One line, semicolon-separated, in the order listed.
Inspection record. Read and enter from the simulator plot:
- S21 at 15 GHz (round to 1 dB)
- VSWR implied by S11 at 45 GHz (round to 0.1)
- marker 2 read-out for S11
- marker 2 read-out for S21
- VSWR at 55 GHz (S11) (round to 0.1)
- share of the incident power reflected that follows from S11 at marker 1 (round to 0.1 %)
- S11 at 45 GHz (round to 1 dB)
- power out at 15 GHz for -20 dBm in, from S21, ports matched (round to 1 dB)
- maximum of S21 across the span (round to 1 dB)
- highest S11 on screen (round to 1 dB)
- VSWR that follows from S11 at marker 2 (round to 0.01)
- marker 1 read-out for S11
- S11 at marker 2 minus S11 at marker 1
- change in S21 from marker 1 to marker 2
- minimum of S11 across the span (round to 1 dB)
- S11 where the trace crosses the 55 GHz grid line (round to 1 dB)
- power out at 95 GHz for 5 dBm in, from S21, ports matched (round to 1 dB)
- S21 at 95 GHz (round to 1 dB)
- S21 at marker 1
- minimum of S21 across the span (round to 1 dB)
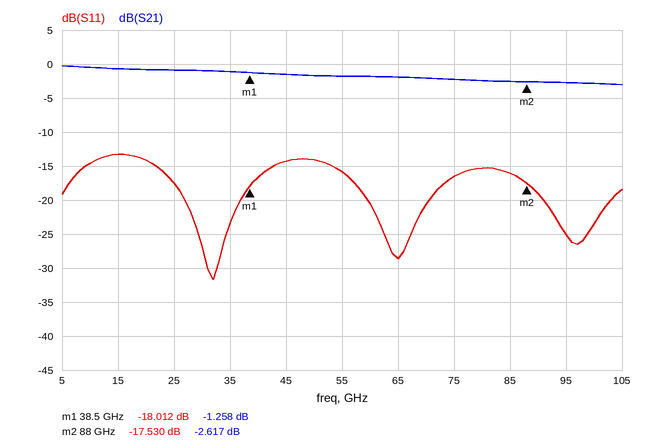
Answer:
-1 dB; 1.5; -17.530 dB; -2.617 dB; 1.4; 1.6 %; -14 dB; -21 dBm; 0 dB; -13 dB; 1.31; -18.012 dB; 0.482 dB; -1.359 dB; -32 dB; -16 dB; 2 dBm; -3 dB; -1.258 dB; -3 dB
